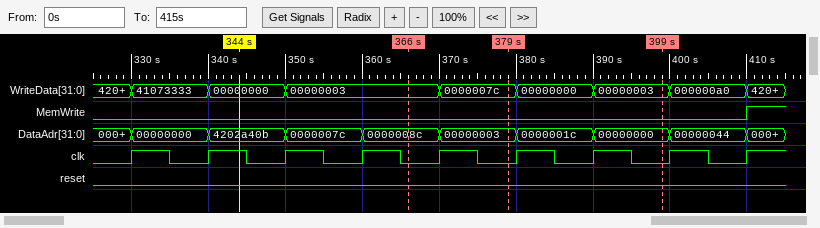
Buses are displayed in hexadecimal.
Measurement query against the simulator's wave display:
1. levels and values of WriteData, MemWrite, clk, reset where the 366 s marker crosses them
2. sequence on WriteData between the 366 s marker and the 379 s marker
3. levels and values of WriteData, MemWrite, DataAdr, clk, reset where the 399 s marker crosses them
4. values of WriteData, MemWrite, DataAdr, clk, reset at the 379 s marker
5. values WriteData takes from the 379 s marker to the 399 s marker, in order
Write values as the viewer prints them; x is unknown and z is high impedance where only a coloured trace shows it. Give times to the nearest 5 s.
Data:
WriteData=00000003, MemWrite=0, clk=0, reset=0
00000003, 0000007c
WriteData=00000003, MemWrite=0, DataAdr=00000000, clk=0, reset=0
WriteData=0000007c, MemWrite=0, DataAdr=00000003, clk=0, reset=0
0000007c, 00000000, 00000003
